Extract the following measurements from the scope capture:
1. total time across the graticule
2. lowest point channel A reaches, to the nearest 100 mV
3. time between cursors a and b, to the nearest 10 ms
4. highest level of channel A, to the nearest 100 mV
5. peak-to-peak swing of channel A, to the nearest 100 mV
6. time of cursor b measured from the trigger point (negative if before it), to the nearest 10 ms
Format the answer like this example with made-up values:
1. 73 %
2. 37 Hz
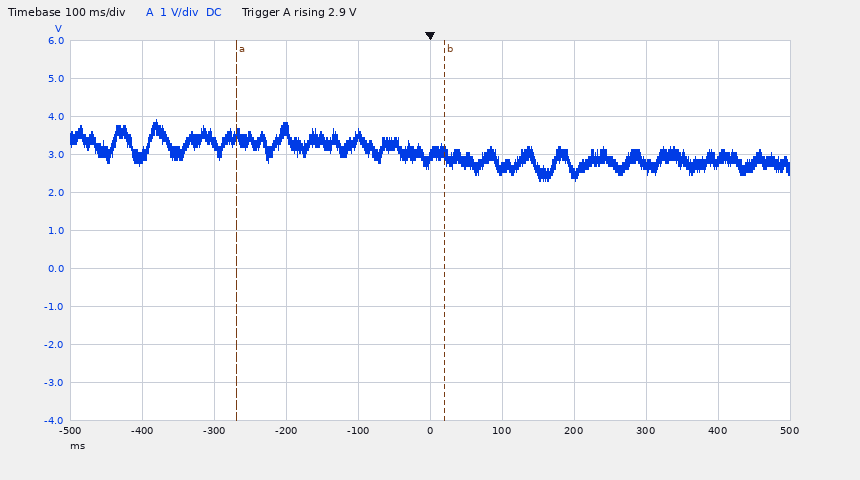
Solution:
1. 1 s
2. 2.3 V
3. 290 ms
4. 3.9 V
5. 1.6 V
6. +20 ms
